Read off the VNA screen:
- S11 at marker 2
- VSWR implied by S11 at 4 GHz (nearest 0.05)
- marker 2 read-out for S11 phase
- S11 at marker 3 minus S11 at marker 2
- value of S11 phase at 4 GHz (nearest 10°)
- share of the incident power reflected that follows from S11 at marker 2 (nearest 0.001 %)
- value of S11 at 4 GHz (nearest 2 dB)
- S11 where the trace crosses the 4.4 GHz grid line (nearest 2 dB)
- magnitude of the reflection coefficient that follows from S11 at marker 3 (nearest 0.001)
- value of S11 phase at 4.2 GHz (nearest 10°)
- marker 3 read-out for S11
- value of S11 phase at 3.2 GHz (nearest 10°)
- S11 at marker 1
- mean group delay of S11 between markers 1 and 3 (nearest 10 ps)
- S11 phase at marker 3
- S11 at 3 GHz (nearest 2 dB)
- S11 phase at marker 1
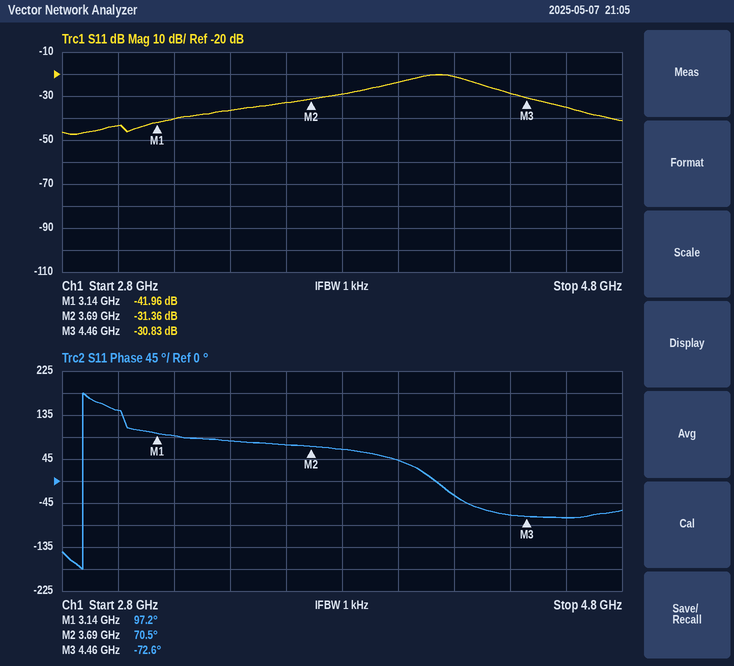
-31.36 dB
1.15
70.5°
0.53 dB
40°
0.073 %
-24 dB
-28 dB
0.029
-30°
-30.83 dB
90°
-41.96 dB
360 ps
-72.6°
-44 dB
97.2°
